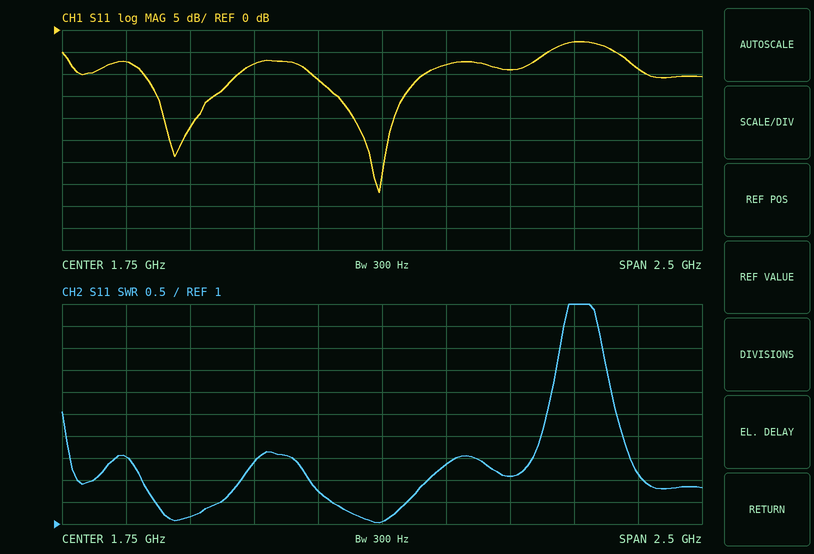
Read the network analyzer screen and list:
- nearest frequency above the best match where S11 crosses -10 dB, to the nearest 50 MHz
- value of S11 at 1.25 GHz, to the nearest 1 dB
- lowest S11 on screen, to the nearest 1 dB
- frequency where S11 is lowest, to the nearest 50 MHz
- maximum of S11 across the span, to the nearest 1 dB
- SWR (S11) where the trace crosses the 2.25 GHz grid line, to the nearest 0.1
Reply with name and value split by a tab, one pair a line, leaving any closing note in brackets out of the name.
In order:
nearest frequency above the best match where S11 crosses -10 dB, to the nearest 50 MHz	1.90 GHz
value of S11 at 1.25 GHz, to the nearest 1 dB	-8 dB
lowest S11 on screen, to the nearest 1 dB	-37 dB
frequency where S11 is lowest, to the nearest 50 MHz	1.75 GHz
maximum of S11 across the span, to the nearest 1 dB	-3 dB
SWR (S11) where the trace crosses the 2.25 GHz grid line, to the nearest 0.1	2.1
